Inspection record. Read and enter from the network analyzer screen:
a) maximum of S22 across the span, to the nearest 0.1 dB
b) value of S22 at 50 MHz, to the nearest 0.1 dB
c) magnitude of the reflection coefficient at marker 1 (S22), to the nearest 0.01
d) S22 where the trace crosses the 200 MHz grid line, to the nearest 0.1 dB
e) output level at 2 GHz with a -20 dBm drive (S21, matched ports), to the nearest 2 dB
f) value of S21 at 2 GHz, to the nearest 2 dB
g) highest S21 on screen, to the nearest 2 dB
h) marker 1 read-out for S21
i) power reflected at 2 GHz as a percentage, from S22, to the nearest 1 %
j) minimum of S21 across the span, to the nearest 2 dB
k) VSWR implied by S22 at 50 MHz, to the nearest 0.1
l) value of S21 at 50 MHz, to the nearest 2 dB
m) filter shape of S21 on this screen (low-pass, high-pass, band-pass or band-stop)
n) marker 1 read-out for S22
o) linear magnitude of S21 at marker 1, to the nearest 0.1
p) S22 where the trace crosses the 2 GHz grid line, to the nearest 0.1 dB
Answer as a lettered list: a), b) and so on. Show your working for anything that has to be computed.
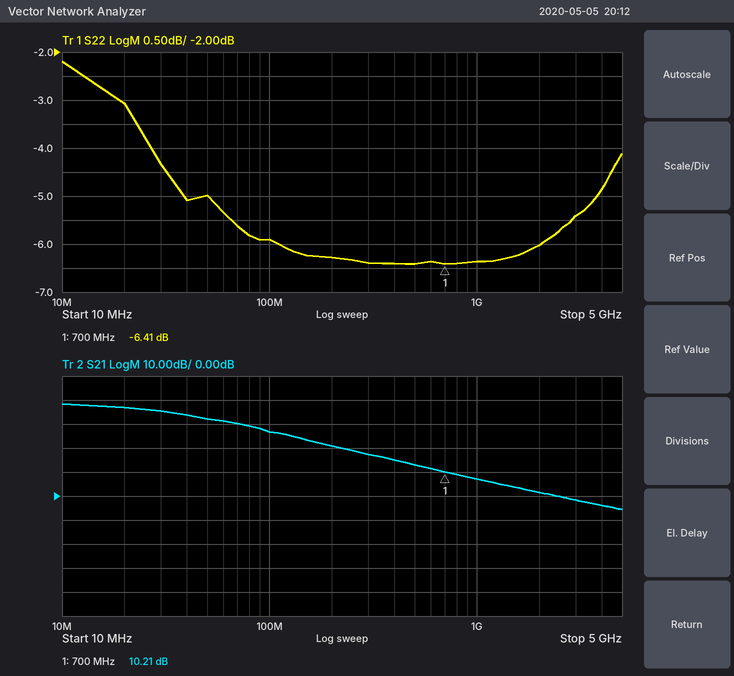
a) -2.2 dB
b) -5.0 dB
c) 10^(-6.41/20) ≈ 0.48
d) -6.3 dB
e) -20 dBm + (2 dB) = -18 dBm
f) 2 dB
g) 38 dB
h) 10.21 dB
i) 10^(-6/10) ≈ 25 %
j) -6 dB
k) |Γ| = 10^(-5/20) = 0.5623; VSWR = (1 + 0.5623)/(1 − 0.5623) ≈ 3.6
l) 32 dB
m) low-pass
n) -6.41 dB
o) 10^(10.21/20) ≈ 3.2
p) -6.0 dB
